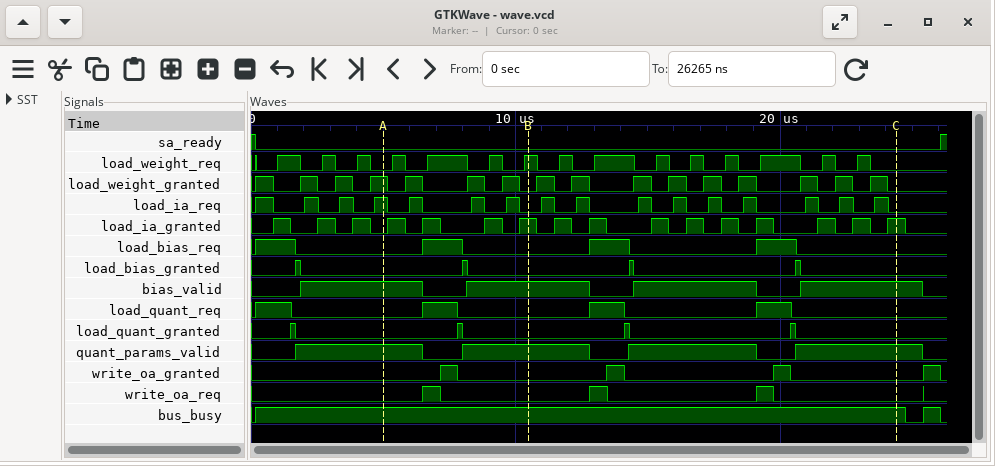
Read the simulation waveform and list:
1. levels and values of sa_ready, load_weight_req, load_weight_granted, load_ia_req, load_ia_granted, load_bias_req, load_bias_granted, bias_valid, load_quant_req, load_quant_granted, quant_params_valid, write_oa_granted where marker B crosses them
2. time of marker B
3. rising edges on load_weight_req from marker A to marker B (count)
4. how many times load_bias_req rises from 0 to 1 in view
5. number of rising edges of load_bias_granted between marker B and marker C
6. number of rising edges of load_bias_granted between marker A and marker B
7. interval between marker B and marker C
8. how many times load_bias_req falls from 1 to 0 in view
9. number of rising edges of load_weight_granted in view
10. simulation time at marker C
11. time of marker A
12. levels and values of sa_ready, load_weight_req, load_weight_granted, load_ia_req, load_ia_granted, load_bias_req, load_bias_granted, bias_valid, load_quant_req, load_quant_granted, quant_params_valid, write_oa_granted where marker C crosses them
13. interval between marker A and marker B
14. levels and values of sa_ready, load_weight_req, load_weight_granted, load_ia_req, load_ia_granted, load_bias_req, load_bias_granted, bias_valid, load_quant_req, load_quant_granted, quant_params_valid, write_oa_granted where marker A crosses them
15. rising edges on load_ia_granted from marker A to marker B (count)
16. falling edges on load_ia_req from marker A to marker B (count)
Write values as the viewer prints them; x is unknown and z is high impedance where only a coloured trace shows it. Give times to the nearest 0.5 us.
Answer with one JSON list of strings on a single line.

["sa_ready=0, load_weight_req=1, load_weight_granted=0, load_ia_req=0, load_ia_granted=1, load_bias_req=0, load_bias_granted=0, bias_valid=1, load_quant_req=0, load_quant_granted=0, quant_params_valid=1, write_oa_granted=0", "10.5 us", "4", "4", "2", "1", "14 us", "4", "16", "24.5 us", "5 us", "sa_ready=0, load_weight_req=0, load_weight_granted=0, load_ia_req=0, load_ia_granted=1, load_bias_req=0, load_bias_granted=0, bias_valid=1, load_quant_req=0, load_quant_granted=0, quant_params_valid=1, write_oa_granted=0", "5.5 us", "sa_ready=0, load_weight_req=0, load_weight_granted=1, load_ia_req=1, load_ia_granted=0, load_bias_req=0, load_bias_granted=0, bias_valid=1, load_quant_req=0, load_quant_granted=0, quant_params_valid=1, write_oa_granted=0", "4", "4"]
